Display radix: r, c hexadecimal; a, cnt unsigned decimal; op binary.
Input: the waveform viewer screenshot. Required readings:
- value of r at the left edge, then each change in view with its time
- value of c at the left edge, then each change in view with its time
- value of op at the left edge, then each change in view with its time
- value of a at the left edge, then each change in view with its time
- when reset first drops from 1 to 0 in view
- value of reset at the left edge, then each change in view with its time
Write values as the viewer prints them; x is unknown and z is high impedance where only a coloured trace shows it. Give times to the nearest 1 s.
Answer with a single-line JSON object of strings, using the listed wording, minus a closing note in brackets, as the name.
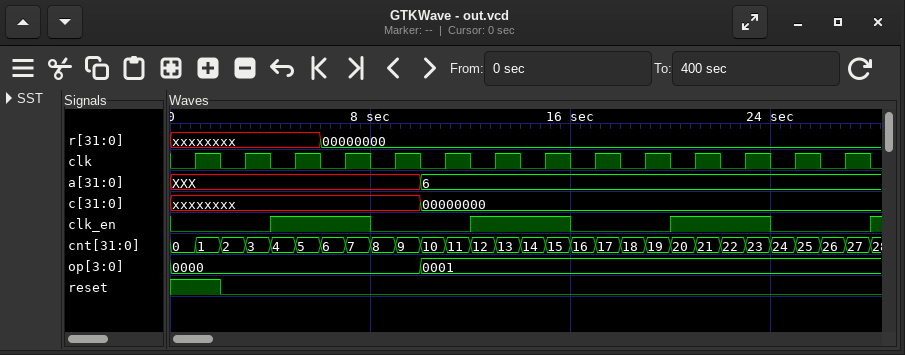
{"value of r at the left edge, then each change in view with its time": "xxxxxxxx, 00000000 at 6 s", "value of c at the left edge, then each change in view with its time": "xxxxxxxx, 00000000 at 10 s", "value of op at the left edge, then each change in view with its time": "0000, 0001 at 10 s", "value of a at the left edge, then each change in view with its time": "XXX, 6 at 10 s", "when reset first drops from 1 to 0 in view": "2 s", "value of reset at the left edge, then each change in view with its time": "1, 0 at 2 s"}
